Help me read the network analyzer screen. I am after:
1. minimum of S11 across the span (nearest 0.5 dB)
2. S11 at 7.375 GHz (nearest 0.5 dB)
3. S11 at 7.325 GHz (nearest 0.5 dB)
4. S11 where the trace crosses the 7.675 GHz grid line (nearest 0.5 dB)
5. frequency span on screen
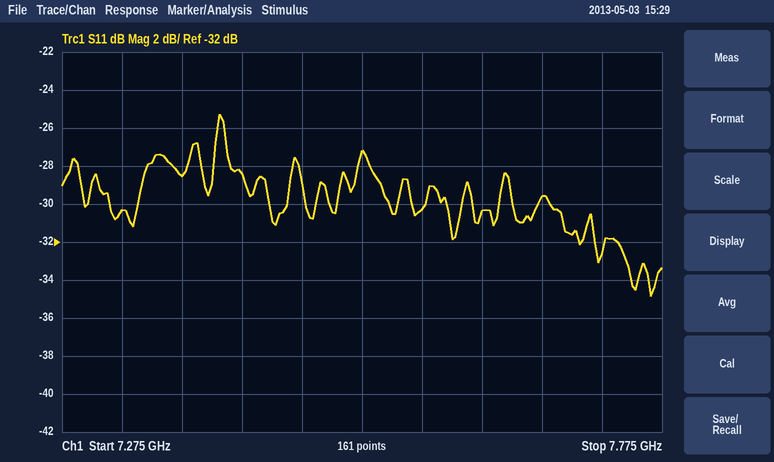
-35.0 dB
-28.5 dB
-30.5 dB
-29.5 dB
500 MHz
